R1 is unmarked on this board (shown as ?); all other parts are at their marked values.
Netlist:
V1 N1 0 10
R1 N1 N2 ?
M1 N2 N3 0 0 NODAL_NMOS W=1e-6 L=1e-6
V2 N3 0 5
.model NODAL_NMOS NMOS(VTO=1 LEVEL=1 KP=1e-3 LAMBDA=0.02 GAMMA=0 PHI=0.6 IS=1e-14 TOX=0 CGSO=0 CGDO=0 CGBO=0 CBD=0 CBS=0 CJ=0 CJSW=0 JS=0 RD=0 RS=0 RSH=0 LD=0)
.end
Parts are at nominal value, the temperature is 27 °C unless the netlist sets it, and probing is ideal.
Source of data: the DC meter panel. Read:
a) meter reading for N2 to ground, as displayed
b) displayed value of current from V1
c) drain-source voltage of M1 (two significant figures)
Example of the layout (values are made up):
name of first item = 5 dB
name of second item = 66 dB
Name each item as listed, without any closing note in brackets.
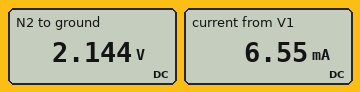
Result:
meter reading for N2 to ground, as displayed = 2.144 V
displayed value of current from V1 = 6.55 mA
drain-source voltage of M1 = 2.1 V
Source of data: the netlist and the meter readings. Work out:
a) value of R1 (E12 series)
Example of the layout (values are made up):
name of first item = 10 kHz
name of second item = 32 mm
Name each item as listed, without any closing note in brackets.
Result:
value of R1 = 1.2 kΩ
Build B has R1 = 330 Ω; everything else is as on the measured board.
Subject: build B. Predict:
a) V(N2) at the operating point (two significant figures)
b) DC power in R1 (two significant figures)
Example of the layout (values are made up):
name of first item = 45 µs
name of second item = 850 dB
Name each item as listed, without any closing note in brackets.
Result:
V(N2) at the operating point = 7.0 V
DC power in R1 = 27 mW
